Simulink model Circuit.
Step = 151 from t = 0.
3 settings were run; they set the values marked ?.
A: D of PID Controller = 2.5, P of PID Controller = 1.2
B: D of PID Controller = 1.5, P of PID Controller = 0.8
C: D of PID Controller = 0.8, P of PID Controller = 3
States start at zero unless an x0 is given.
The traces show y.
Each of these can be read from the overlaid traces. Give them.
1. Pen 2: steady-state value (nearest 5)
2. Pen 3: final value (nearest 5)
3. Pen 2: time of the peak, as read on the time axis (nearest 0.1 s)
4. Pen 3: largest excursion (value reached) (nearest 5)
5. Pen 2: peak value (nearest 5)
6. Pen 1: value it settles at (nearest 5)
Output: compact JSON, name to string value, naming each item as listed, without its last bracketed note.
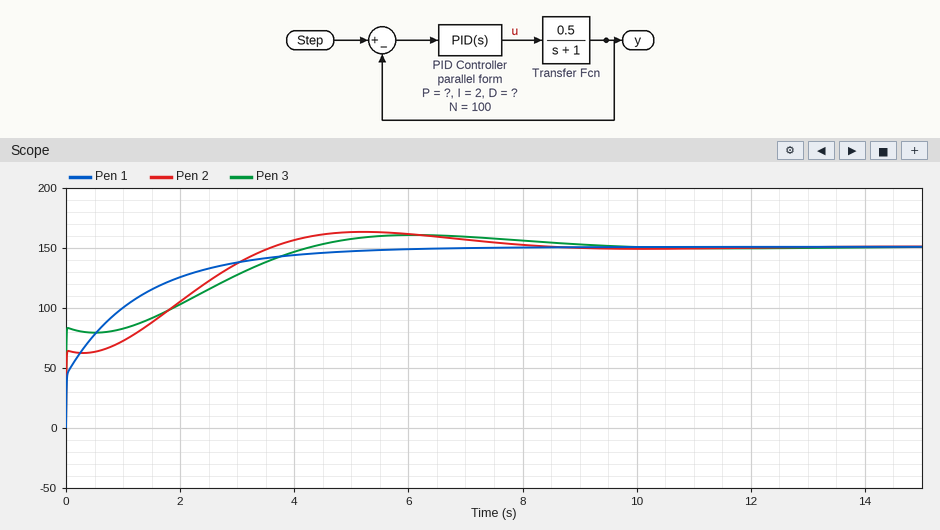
{"Pen 2: steady-state value": "150", "Pen 3: final value": "150", "Pen 2: time of the peak, as read on the time axis": "5.2 s", "Pen 3: largest excursion (value reached)": "160", "Pen 2: peak value": "165", "Pen 1: value it settles at": "150"}
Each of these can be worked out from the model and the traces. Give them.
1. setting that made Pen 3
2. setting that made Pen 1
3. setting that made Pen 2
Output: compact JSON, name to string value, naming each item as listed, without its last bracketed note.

{"setting that made Pen 3": "A", "setting that made Pen 1": "C", "setting that made Pen 2": "B"}
